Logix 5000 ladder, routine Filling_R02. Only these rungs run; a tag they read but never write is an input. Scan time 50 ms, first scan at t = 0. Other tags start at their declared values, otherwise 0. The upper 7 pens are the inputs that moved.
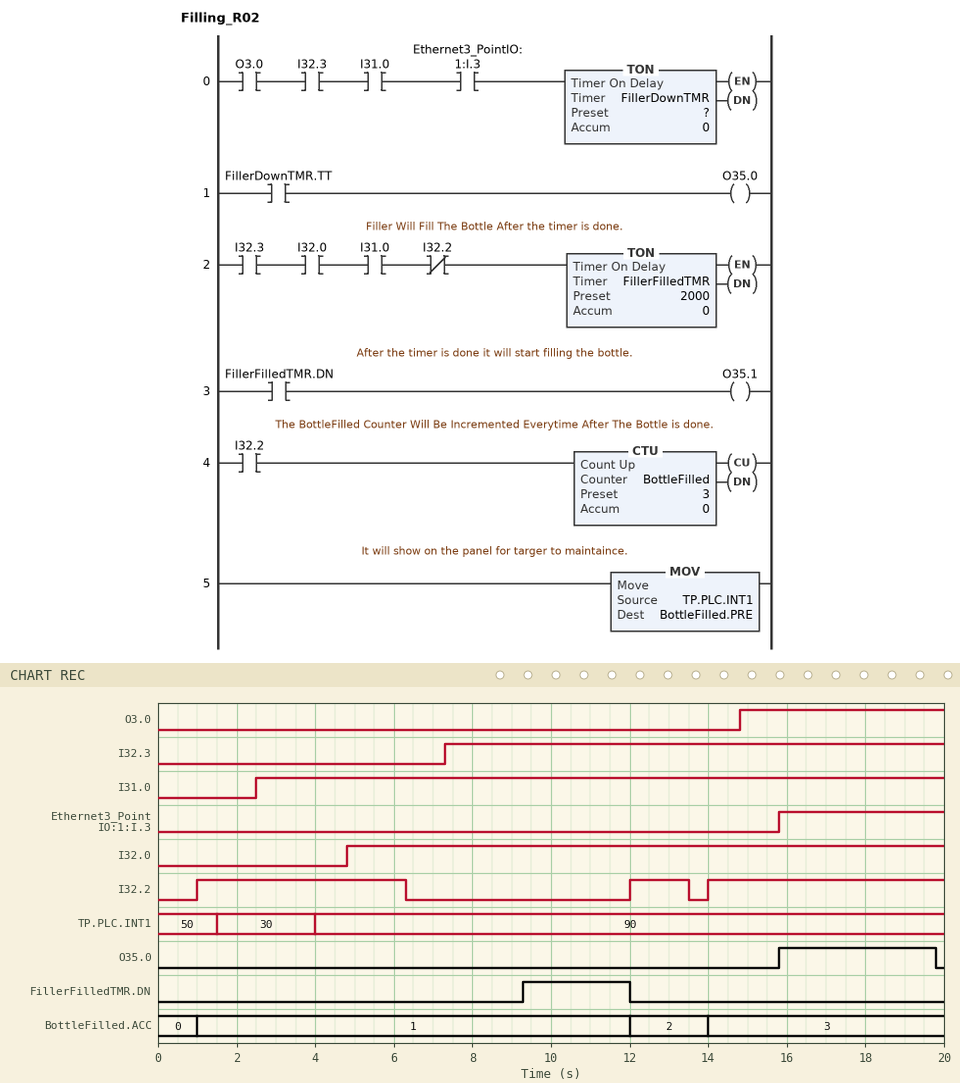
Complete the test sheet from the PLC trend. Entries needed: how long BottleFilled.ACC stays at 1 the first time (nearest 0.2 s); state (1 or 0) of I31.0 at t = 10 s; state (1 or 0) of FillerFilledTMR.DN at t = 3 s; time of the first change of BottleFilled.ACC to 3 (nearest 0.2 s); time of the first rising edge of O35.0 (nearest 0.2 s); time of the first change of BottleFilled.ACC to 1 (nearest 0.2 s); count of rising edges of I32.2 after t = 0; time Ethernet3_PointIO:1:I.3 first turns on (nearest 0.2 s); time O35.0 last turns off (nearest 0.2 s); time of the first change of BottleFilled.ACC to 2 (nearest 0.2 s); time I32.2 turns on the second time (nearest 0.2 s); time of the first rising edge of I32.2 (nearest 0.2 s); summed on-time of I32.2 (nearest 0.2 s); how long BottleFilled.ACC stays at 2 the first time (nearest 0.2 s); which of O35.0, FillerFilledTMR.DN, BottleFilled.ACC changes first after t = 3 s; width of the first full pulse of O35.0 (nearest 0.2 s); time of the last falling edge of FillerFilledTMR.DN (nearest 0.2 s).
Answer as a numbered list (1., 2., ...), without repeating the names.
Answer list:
1. 11.0 s
2. 1
3. 0
4. 14.0 s
5. 15.8 s
6. 1.0 s
7. 3
8. 15.8 s
9. 19.8 s
10. 12.0 s
11. 12.0 s
12. 1.0 s
13. 12.8 s
14. 2.0 s
15. FillerFilledTMR.DN
16. 4.0 s
17. 12.0 s
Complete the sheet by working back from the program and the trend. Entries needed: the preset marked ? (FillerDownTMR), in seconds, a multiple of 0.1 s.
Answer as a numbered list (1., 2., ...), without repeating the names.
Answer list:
1. 4.0 s
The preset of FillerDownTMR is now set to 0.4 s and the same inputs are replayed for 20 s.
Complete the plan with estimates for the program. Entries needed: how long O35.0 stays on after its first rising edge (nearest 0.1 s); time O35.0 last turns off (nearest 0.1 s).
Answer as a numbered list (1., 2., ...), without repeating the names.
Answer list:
1. 0.4 s
2. 16.2 s
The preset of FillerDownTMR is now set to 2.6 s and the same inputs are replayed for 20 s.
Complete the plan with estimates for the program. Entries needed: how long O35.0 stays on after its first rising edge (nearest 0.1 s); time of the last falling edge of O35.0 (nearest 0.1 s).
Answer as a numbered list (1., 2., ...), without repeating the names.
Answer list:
1. 2.6 s
2. 18.4 s
